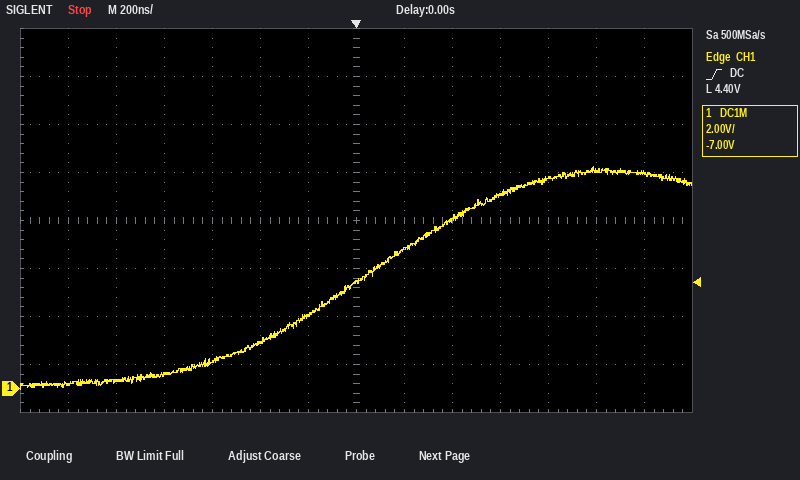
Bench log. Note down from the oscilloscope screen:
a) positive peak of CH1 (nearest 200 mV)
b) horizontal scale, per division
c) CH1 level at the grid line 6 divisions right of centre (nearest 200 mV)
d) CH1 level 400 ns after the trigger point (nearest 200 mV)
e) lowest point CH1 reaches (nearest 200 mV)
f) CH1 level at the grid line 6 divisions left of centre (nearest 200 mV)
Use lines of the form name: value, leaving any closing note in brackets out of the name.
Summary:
positive peak of CH1: 9.2 V
horizontal scale, per division: 200 ns
CH1 level at the grid line 6 divisions right of centre: 9.0 V
CH1 level 400 ns after the trigger point: 7.0 V
lowest point CH1 reaches: 0.0 V
CH1 level at the grid line 6 divisions left of centre: 200 mV
